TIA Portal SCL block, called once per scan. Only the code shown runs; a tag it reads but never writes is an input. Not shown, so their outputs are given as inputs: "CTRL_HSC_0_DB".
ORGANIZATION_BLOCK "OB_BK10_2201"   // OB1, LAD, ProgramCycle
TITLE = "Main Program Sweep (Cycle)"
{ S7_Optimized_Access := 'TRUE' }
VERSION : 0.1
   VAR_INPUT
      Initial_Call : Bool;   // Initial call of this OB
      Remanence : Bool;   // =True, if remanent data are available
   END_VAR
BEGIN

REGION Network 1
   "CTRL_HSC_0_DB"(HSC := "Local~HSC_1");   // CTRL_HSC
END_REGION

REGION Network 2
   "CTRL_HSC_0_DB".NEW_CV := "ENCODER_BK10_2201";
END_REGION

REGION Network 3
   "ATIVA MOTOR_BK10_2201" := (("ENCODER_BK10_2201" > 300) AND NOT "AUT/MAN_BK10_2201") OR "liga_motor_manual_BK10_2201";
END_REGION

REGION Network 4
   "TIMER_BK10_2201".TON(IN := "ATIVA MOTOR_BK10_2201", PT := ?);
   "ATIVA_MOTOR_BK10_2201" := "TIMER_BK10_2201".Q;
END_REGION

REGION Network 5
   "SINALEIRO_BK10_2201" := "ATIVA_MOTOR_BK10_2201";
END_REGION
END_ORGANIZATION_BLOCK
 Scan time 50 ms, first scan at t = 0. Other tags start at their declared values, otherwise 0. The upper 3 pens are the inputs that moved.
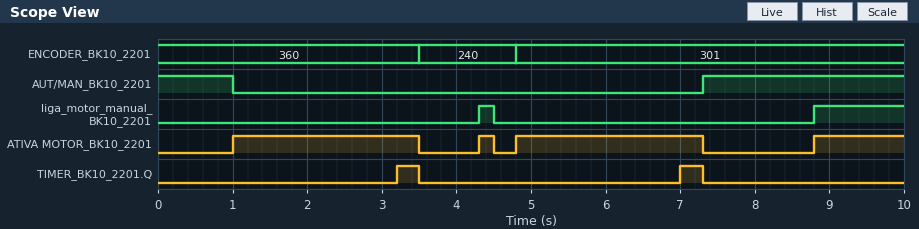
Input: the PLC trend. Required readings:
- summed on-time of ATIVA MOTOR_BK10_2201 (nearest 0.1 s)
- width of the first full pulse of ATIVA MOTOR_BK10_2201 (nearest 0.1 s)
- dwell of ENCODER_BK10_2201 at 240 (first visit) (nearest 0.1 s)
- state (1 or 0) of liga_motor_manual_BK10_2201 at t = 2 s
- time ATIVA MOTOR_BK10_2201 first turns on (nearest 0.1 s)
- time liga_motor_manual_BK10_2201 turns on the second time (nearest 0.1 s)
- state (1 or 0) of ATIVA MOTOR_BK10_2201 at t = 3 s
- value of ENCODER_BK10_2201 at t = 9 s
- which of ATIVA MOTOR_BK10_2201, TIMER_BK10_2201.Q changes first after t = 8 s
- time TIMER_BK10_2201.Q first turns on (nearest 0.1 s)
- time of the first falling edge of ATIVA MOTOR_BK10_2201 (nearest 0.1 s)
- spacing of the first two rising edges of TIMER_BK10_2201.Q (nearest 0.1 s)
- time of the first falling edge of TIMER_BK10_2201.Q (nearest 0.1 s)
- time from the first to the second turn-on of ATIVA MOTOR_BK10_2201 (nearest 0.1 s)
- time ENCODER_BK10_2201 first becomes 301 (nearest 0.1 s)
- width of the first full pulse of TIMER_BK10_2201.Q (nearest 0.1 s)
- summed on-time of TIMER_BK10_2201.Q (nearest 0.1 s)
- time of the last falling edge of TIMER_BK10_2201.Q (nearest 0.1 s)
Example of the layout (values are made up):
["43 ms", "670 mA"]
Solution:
["6.4 s", "2.5 s", "1.3 s", "0", "1.0 s", "8.8 s", "1", "301", "ATIVA MOTOR_BK10_2201", "3.2 s", "3.5 s", "3.8 s", "3.5 s", "3.3 s", "4.8 s", "0.3 s", "0.6 s", "7.3 s"]
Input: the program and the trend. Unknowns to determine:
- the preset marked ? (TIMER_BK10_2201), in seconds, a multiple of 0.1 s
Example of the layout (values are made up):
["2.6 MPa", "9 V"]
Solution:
["2.2 s"]
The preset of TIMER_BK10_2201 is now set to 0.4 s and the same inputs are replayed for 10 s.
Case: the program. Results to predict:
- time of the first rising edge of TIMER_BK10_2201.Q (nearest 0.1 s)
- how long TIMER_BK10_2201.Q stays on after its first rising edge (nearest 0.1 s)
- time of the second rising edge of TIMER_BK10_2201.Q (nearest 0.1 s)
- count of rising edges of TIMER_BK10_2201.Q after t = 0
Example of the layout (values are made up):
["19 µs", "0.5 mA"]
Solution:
["1.4 s", "2.1 s", "5.2 s", "3"]
